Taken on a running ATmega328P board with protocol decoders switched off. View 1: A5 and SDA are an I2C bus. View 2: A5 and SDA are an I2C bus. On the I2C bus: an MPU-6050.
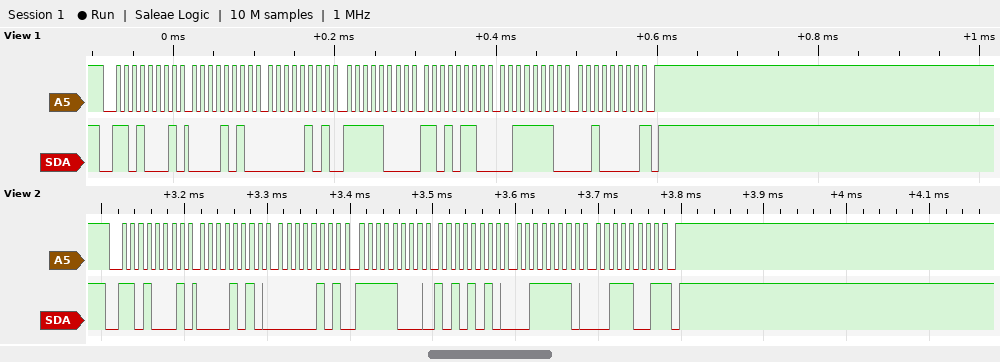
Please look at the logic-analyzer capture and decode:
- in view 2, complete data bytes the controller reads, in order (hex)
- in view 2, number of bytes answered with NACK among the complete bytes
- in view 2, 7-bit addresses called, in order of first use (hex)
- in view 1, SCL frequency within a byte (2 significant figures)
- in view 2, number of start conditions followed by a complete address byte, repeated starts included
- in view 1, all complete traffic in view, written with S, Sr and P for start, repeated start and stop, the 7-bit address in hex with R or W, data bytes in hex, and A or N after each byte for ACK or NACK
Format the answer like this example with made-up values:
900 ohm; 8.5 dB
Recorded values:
0A 05 F8 AA 3E 39; 1; 0x68; 100 kHz; 1; S 68R A 0A A 05 A F8 A D6 A 3E A 20 N P
